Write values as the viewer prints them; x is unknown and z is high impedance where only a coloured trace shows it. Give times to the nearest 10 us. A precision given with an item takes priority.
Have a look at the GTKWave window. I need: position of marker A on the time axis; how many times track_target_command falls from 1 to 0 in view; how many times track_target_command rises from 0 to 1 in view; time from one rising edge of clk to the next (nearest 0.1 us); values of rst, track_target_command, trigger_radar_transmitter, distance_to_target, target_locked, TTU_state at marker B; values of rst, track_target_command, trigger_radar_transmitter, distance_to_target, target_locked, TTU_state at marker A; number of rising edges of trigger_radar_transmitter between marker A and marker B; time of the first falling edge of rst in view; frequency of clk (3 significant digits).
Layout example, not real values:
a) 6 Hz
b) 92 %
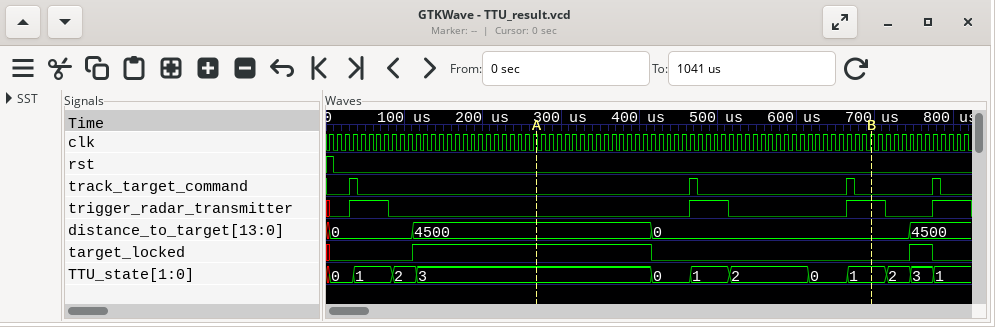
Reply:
a) 270 us
b) 4
c) 4
d) 10 us
e) rst=0, track_target_command=0, trigger_radar_transmitter=1, distance_to_target=0, target_locked=0, TTU_state=1
f) rst=0, track_target_command=0, trigger_radar_transmitter=0, distance_to_target=4500, target_locked=1, TTU_state=3
g) 2
h) 10 us
i) 100 kHz
